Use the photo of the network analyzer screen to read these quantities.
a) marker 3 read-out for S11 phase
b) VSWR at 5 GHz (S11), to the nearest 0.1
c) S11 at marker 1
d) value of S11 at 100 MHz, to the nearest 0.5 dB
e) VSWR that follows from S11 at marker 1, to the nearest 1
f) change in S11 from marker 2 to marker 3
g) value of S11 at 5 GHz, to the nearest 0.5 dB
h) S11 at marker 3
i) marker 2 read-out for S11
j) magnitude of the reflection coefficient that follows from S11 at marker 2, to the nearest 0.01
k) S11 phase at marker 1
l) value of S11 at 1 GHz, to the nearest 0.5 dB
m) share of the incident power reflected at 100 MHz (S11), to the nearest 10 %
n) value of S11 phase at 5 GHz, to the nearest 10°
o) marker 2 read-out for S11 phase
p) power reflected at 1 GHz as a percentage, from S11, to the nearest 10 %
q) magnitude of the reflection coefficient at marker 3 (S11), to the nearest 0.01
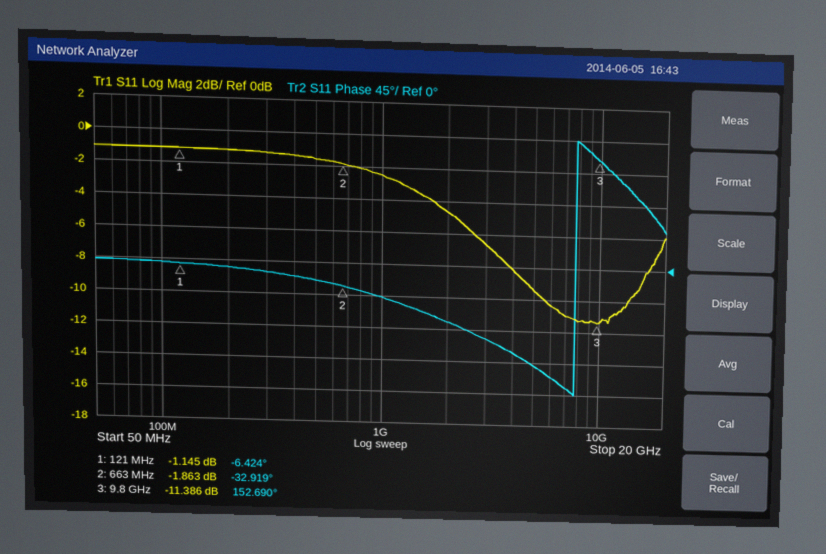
152.690°
2.0
-1.145 dB
-1.0 dB
15
-9.523 dB
-9.5 dB
-11.386 dB
-1.863 dB
0.81
-6.424°
-2.5 dB
80 %
-140°
-32.919°
60 %
0.27
